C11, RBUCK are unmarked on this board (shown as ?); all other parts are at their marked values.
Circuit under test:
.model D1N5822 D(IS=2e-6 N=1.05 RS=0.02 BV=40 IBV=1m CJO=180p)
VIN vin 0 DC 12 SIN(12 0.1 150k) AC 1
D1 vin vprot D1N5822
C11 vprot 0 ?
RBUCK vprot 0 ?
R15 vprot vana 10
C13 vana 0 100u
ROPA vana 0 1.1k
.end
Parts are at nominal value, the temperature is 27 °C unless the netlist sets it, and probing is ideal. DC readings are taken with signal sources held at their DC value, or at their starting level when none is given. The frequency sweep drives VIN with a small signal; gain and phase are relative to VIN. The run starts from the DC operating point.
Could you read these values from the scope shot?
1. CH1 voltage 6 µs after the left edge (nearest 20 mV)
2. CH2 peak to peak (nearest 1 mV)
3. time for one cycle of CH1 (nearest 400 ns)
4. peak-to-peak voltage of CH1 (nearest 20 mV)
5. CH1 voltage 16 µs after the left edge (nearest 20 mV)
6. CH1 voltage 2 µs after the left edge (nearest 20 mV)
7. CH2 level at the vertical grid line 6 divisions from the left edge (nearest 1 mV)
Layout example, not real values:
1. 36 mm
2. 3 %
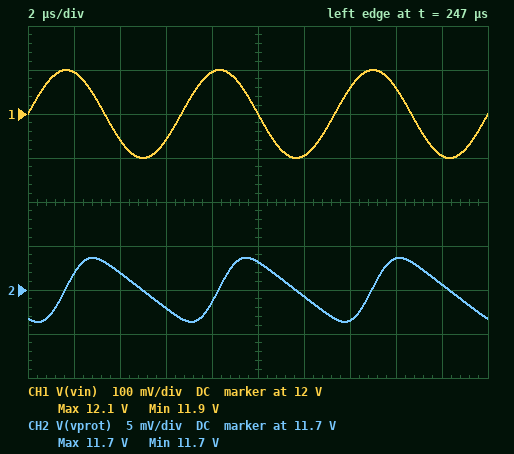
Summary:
1. 11.94 V
2. 7 mV
3. 6.8 µs
4. 200 mV
5. 12.06 V
6. 12.10 V
7. 11.699 V
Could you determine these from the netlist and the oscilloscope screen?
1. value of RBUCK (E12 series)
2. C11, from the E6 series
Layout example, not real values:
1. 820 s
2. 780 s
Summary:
1. 27 Ω
2. 220 µF
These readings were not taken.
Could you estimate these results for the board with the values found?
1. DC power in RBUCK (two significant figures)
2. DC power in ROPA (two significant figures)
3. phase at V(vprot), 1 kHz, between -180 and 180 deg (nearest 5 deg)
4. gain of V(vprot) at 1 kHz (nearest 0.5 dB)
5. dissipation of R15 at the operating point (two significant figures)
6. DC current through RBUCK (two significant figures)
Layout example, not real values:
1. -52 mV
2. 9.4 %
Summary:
1. 5.0 W
2. 120 mW
3. -5 deg
4. 0 dB
5. 1.1 mW
6. 430 mA
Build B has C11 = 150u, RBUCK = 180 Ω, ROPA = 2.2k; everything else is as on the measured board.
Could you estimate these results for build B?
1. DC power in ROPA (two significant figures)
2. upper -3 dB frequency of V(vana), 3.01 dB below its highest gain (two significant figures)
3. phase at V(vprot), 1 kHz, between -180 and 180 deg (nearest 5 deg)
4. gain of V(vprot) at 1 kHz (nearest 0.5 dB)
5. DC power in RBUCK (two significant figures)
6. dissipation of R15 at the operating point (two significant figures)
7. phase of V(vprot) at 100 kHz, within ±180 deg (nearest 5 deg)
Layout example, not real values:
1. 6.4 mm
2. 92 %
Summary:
1. 62 mW
2. 150 Hz
3. -20 deg
4. -1.0 dB
5. 760 mW
6. 280 µW
7. -90 deg
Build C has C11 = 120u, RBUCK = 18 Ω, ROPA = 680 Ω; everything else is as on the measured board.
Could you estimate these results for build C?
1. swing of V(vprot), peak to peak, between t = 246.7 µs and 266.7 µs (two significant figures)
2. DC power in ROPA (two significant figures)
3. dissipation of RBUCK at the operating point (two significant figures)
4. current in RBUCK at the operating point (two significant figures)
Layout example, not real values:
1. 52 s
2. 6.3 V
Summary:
1. 19 mV
2. 190 mW
3. 7.5 W
4. 650 mA
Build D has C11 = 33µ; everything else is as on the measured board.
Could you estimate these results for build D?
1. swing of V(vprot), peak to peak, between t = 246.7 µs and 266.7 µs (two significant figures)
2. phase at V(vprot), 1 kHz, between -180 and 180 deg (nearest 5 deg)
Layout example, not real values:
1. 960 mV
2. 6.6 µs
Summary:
1. 48 mV
2. 0 deg
